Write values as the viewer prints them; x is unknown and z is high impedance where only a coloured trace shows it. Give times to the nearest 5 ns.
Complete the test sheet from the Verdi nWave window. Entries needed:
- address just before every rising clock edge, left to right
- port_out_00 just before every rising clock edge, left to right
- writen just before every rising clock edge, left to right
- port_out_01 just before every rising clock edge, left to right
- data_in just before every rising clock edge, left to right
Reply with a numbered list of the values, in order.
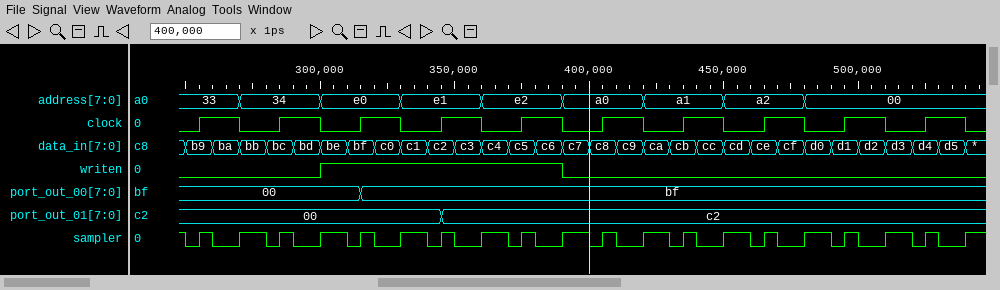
1. 33, 34, e0, e1, e2, a0, a1, a2, 00, 00
2. 00, 00, 00, bf, bf, bf, bf, bf, bf, bf
3. 0 0 1 1 1 0 0 0 0 0
4. 00, 00, 00, 00, c2, c2, c2, c2, c2, c2
5. b9, bc, bf, c2, c5, c8, cb, ce, d1, d4
